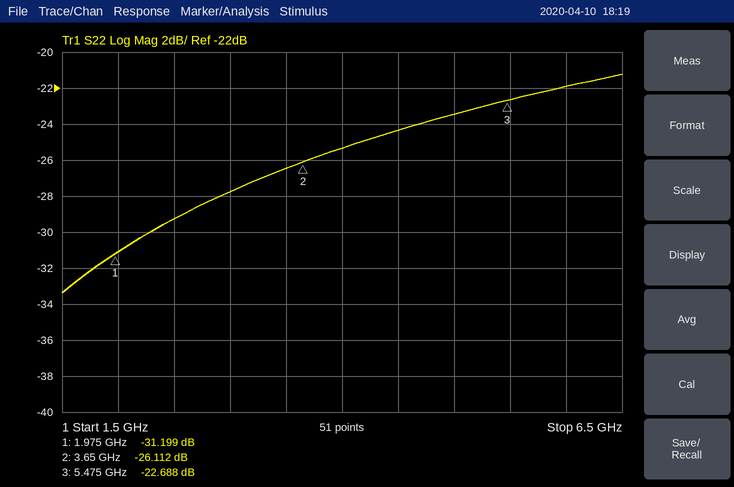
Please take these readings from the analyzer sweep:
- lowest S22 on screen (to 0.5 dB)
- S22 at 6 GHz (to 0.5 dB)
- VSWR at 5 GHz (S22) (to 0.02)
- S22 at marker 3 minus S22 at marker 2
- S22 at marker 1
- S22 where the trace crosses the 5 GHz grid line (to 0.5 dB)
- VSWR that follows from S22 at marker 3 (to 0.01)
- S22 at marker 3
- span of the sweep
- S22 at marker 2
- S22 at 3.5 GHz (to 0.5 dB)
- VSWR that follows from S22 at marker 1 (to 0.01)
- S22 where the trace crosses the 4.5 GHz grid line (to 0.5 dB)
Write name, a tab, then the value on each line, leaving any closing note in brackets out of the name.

lowest S22 on screen	-33.5 dB
S22 at 6 GHz	-22.0 dB
VSWR at 5 GHz (S22)	1.14
S22 at marker 3 minus S22 at marker 2	3.424 dB
S22 at marker 1	-31.199 dB
S22 where the trace crosses the 5 GHz grid line	-23.5 dB
VSWR that follows from S22 at marker 3	1.16
S22 at marker 3	-22.688 dB
span of the sweep	5 GHz
S22 at marker 2	-26.112 dB
S22 at 3.5 GHz	-26.5 dB
VSWR that follows from S22 at marker 1	1.06
S22 where the trace crosses the 4.5 GHz grid line	-24.5 dB
